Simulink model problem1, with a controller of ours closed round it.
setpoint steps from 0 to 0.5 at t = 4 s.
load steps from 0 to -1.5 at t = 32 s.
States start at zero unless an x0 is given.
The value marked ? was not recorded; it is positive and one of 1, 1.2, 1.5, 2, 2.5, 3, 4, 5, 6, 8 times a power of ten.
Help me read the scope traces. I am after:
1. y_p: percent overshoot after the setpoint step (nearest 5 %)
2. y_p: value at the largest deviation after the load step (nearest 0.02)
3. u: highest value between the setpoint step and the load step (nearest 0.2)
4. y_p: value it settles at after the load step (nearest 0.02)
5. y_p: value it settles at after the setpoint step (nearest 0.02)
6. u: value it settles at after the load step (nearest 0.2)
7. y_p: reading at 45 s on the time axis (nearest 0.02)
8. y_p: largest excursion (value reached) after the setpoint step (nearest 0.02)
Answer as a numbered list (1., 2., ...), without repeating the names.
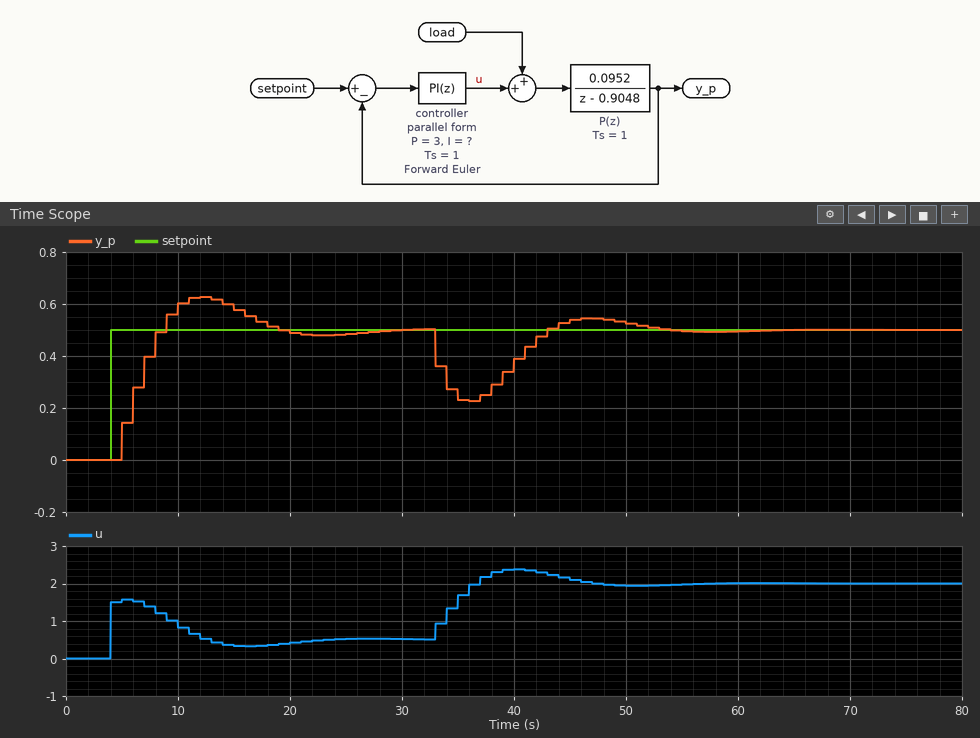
1. 25 %
2. 0.22
3. 1.6
4. 0.50
5. 0.50
6. 2.0
7. 0.54
8. 0.62
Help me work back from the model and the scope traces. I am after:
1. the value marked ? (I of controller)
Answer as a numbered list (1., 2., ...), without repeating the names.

1. 1
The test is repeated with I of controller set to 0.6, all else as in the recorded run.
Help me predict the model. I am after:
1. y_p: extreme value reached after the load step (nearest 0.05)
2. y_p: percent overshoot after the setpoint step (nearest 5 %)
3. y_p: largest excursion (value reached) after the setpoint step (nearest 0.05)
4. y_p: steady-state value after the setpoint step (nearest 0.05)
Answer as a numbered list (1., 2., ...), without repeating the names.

1. 0.20
2. 10 %
3. 0.55
4. 0.50
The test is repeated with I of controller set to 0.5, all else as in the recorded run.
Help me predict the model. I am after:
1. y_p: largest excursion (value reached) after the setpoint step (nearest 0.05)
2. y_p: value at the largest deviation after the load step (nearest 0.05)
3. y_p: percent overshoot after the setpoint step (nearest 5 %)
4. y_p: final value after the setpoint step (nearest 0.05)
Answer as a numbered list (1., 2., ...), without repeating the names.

1. 0.55
2. 0.20
3. 10 %
4. 0.50
